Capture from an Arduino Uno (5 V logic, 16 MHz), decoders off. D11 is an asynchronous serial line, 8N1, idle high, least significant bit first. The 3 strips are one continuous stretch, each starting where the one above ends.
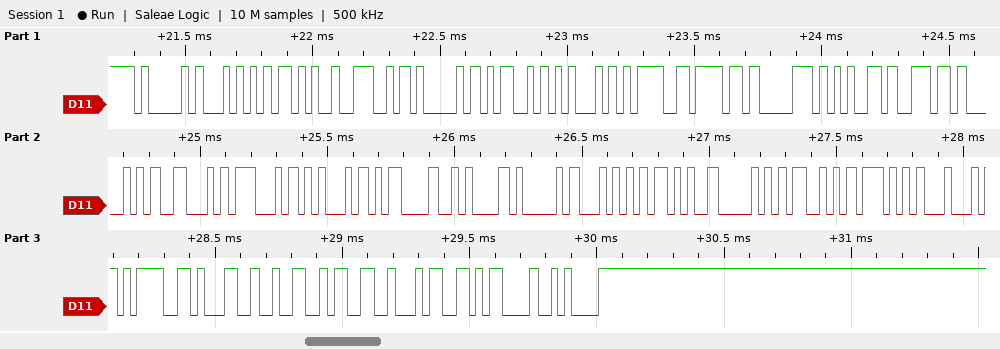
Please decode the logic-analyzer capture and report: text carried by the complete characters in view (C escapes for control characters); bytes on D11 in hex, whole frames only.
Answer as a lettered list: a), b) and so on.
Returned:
a) "AT+NAME=openPFGE\r\nAT+PSWD=1234\r\n"
b) 41 54 2B 4E 41 4D 45 3D 6F 70 65 6E 50 46 47 45 0D 0A 41 54 2B 50 53 57 44 3D 31 32 33 34 0D 0A
